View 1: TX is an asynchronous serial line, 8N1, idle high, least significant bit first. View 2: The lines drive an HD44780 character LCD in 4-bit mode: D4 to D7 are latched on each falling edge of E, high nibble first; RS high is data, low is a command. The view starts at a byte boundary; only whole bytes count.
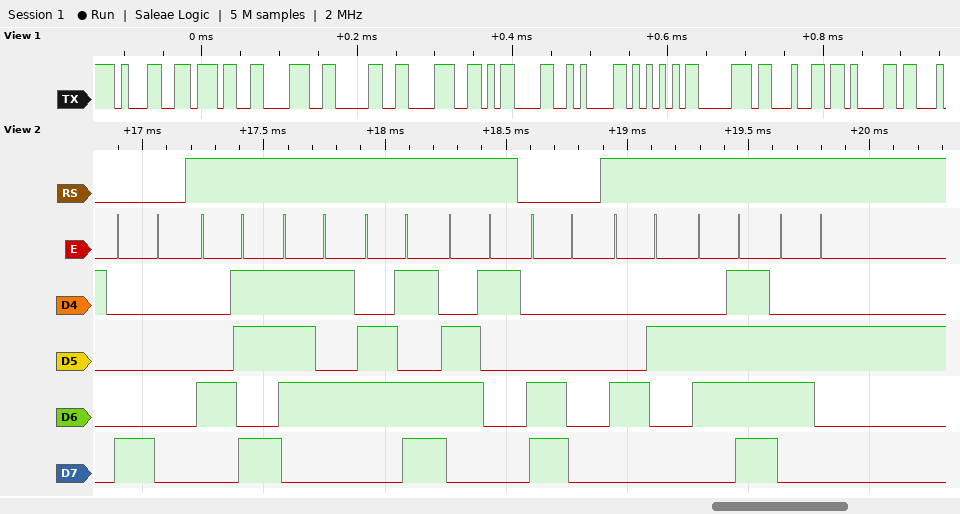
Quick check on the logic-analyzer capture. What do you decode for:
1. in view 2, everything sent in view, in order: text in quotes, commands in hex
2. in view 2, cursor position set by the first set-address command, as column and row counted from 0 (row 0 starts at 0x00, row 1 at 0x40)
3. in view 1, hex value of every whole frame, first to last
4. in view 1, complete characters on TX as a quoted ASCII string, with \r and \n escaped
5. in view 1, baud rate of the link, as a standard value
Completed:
0x80 "Kuma" 0xC0 "Bob"
column 0, row 0
31 37 38 30 38 0D 0A 55 70 64 61
"17808\r\nUpda"
115200 baud
